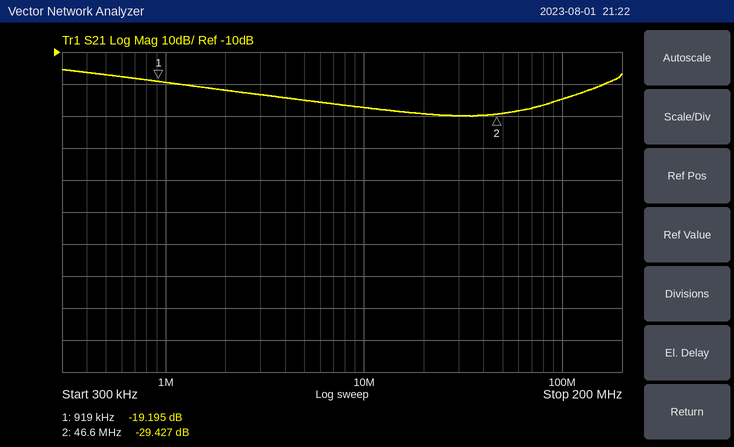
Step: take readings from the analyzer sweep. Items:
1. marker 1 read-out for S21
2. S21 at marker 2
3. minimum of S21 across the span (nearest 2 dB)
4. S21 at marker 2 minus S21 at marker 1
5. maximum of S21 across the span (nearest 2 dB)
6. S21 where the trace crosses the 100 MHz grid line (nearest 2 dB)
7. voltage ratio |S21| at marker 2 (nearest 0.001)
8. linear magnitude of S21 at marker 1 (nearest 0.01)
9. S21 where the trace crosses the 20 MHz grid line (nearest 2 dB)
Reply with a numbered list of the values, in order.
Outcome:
1. -19.195 dB
2. -29.427 dB
3. -30 dB
4. -10.232 dB
5. -16 dB
6. -24 dB
7. 0.034
8. 0.11
9. -30 dB
